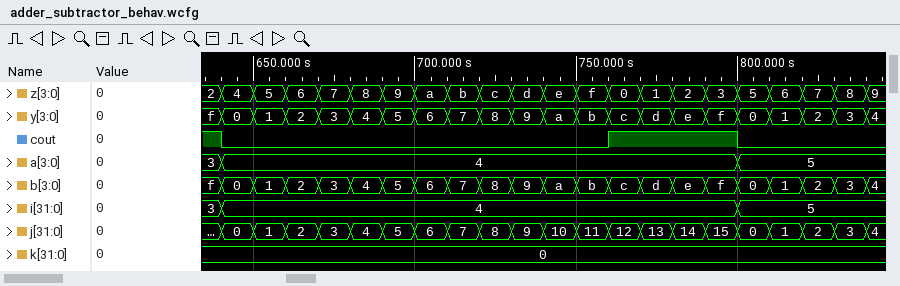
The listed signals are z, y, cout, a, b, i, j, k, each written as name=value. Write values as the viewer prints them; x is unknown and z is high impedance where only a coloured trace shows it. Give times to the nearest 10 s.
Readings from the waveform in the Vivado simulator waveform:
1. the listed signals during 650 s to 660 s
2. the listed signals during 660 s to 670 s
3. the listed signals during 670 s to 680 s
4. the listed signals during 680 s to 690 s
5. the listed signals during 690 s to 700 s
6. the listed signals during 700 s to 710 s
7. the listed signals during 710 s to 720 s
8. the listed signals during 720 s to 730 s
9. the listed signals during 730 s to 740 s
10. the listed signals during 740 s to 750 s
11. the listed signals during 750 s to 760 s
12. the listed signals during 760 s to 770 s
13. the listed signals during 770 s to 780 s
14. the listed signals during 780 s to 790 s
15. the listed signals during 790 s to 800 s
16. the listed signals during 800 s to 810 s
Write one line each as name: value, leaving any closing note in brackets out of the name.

the listed signals during 650 s to 660 s: z=5, y=1, cout=0, a=4, b=1, i=4, j=1, k=0
the listed signals during 660 s to 670 s: z=6, y=2, cout=0, a=4, b=2, i=4, j=2, k=0
the listed signals during 670 s to 680 s: z=7, y=3, cout=0, a=4, b=3, i=4, j=3, k=0
the listed signals during 680 s to 690 s: z=8, y=4, cout=0, a=4, b=4, i=4, j=4, k=0
the listed signals during 690 s to 700 s: z=9, y=5, cout=0, a=4, b=5, i=4, j=5, k=0
the listed signals during 700 s to 710 s: z=a, y=6, cout=0, a=4, b=6, i=4, j=6, k=0
the listed signals during 710 s to 720 s: z=b, y=7, cout=0, a=4, b=7, i=4, j=7, k=0
the listed signals during 720 s to 730 s: z=c, y=8, cout=0, a=4, b=8, i=4, j=8, k=0
the listed signals during 730 s to 740 s: z=d, y=9, cout=0, a=4, b=9, i=4, j=9, k=0
the listed signals during 740 s to 750 s: z=e, y=a, cout=0, a=4, b=a, i=4, j=10, k=0
the listed signals during 750 s to 760 s: z=f, y=b, cout=0, a=4, b=b, i=4, j=11, k=0
the listed signals during 760 s to 770 s: z=0, y=c, cout=1, a=4, b=c, i=4, j=12, k=0
the listed signals during 770 s to 780 s: z=1, y=d, cout=1, a=4, b=d, i=4, j=13, k=0
the listed signals during 780 s to 790 s: z=2, y=e, cout=1, a=4, b=e, i=4, j=14, k=0
the listed signals during 790 s to 800 s: z=3, y=f, cout=1, a=4, b=f, i=4, j=15, k=0
the listed signals during 800 s to 810 s: z=5, y=0, cout=0, a=5, b=0, i=5, j=0, k=0
